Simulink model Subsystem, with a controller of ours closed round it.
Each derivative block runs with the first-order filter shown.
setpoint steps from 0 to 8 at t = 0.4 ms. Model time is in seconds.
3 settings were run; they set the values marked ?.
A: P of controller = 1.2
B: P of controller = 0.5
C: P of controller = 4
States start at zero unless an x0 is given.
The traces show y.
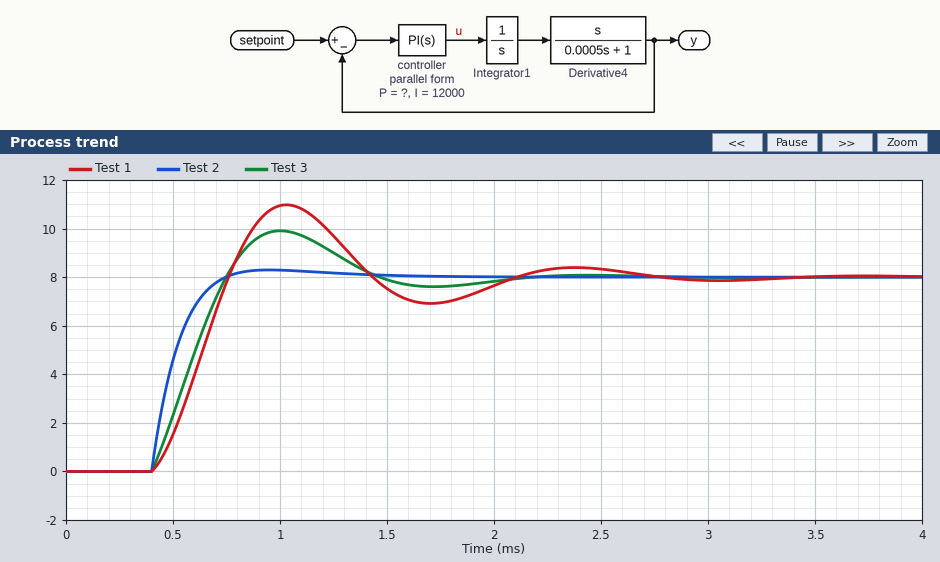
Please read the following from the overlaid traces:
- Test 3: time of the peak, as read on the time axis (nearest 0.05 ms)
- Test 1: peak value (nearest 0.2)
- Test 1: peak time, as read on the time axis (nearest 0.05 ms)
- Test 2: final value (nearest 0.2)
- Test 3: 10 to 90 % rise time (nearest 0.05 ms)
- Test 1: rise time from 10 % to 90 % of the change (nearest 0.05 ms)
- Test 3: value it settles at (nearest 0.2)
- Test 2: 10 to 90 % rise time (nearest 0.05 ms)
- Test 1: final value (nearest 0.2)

1.00 ms
11.0
1.05 ms
8.0
0.25 ms
0.25 ms
8.0
0.20 ms
8.0
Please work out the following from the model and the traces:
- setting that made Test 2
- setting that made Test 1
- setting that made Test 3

C
B
A
